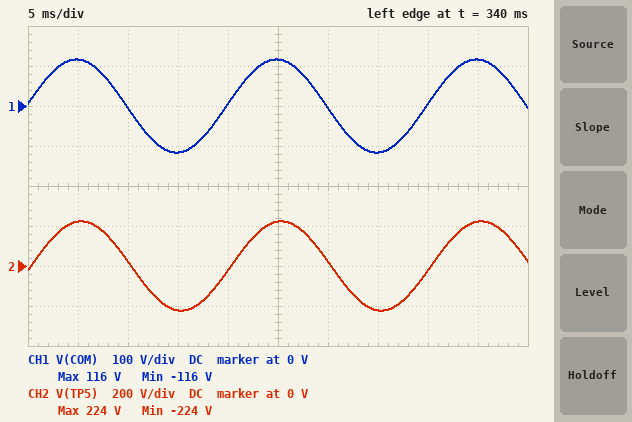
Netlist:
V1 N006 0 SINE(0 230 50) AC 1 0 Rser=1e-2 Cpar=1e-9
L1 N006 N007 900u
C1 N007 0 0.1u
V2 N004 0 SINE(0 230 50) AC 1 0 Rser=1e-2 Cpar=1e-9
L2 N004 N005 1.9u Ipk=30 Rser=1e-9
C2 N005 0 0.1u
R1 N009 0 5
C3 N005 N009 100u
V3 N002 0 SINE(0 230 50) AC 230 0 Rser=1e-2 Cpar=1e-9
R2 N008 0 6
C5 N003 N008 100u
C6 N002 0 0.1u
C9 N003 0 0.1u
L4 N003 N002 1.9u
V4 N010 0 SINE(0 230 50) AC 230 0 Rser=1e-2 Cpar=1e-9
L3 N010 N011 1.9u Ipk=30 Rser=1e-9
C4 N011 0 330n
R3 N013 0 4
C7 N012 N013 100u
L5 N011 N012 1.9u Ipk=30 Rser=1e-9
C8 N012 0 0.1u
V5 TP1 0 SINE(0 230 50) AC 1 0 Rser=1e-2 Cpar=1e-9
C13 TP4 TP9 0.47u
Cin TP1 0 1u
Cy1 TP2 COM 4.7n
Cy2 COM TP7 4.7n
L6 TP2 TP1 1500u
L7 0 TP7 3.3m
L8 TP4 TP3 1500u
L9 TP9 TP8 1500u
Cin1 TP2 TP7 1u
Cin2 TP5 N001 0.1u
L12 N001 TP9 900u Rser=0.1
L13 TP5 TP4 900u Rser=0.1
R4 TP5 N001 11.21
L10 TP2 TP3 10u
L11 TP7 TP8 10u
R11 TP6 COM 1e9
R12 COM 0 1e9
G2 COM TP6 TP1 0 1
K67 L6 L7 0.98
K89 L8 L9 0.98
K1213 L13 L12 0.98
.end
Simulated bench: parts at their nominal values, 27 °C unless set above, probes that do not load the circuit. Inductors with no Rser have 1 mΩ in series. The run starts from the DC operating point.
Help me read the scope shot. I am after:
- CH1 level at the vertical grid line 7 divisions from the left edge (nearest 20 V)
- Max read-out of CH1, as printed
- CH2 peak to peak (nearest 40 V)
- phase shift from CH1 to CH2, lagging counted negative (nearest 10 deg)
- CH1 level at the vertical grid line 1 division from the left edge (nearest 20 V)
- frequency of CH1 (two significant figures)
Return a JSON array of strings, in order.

["-120 V", "116 V", "440 V", "-10 deg", "120 V", "50 Hz"]
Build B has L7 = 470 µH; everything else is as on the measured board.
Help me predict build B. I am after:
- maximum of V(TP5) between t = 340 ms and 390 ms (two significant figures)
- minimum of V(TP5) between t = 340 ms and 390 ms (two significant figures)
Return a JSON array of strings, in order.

["230 V", "-230 V"]
